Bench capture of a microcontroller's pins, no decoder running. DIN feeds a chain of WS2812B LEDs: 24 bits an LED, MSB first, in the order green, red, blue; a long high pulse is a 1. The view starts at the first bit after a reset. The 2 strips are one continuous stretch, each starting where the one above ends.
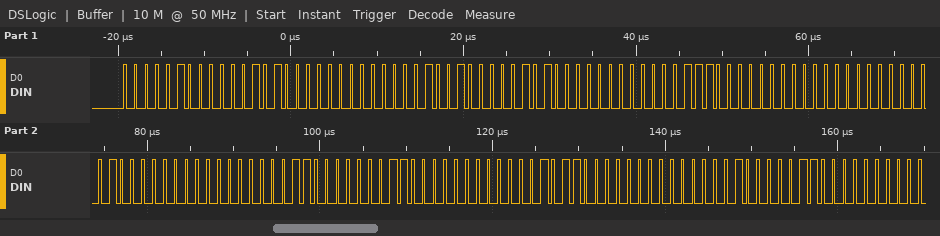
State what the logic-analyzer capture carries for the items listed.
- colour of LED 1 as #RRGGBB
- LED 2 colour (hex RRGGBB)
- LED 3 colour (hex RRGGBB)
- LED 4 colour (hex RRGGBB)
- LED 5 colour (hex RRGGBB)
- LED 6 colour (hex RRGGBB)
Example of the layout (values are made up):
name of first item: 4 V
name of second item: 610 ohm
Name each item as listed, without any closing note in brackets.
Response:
colour of LED 1 as #RRGGBB: #0A0400
LED 2 colour: #050900
LED 3 colour: #000E00
LED 4 colour: #000806
LED 5 colour: #00030B
LED 6 colour: #02000C
